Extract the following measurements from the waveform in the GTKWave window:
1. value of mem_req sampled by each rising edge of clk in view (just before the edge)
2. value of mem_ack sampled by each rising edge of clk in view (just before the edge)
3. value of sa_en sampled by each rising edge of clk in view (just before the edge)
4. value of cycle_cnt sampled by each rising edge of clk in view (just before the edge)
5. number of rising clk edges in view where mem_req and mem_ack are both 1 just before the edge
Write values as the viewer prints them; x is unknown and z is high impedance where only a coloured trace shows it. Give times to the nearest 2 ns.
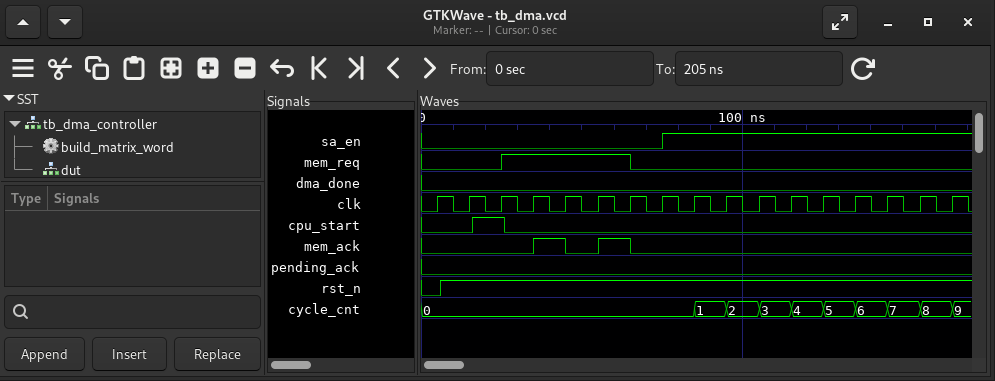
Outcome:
0 0 0 1 1 1 1 0 0 0 0 0 0 0 0 0 0
0 0 0 0 1 0 1 0 0 0 0 0 0 0 0 0 0
0 0 0 0 0 0 0 0 1 1 1 1 1 1 1 1 1
0, 0, 0, 0, 0, 0, 0, 0, 0, 1, 2, 3, 4, 5, 6, 7, 8
2
